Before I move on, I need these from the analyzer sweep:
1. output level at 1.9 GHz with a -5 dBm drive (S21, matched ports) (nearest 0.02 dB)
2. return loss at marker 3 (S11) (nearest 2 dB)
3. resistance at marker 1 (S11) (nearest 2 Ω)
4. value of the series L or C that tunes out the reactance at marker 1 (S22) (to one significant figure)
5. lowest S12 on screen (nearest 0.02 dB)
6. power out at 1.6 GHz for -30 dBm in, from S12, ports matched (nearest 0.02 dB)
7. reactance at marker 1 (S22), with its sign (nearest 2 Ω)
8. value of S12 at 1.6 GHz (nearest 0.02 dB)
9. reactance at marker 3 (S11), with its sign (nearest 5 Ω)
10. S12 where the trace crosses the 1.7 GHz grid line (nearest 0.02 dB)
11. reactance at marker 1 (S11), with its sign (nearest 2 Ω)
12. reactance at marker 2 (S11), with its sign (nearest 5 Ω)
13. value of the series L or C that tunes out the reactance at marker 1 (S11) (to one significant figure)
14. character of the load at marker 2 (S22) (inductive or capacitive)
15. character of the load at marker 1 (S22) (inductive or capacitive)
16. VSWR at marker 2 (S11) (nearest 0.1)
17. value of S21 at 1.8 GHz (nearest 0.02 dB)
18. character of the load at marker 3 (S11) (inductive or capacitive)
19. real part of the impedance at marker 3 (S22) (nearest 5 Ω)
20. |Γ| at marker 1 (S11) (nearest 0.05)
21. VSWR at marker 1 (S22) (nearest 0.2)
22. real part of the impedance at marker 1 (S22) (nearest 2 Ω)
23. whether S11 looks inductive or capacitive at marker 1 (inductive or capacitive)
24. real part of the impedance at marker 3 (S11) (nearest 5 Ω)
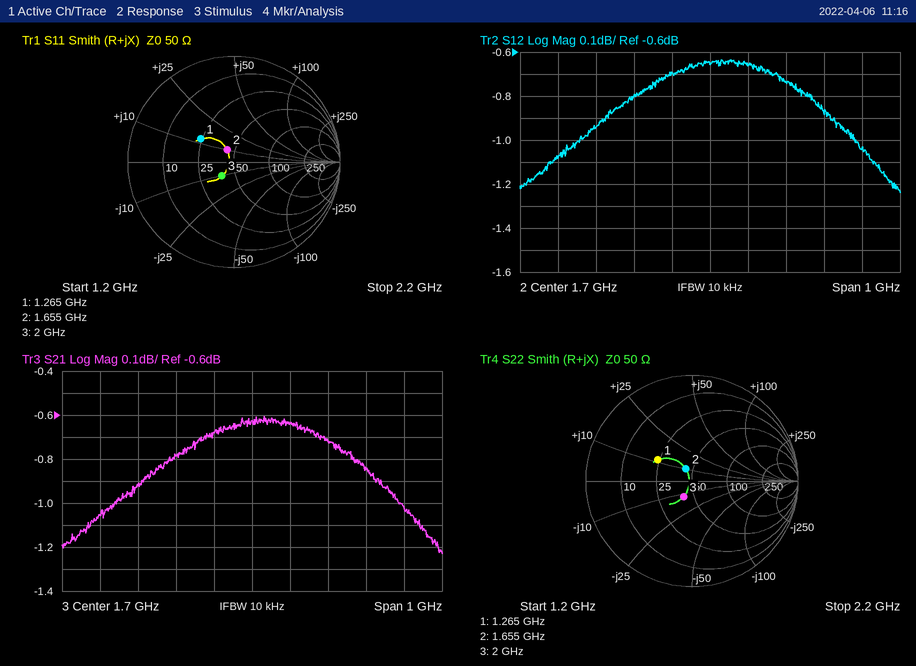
-5.72 dBm
16 dB
24 Ω
10 pF
-1.24 dB
-30.70 dBm
+12 Ω
-0.70 dB
-10 Ω
-0.66 dB
+12 Ω
+10 Ω
10 pF
inductive
inductive
1.3
-0.64 dB
capacitive
40 Ω
0.40
2.2
24 Ω
inductive
40 Ω
